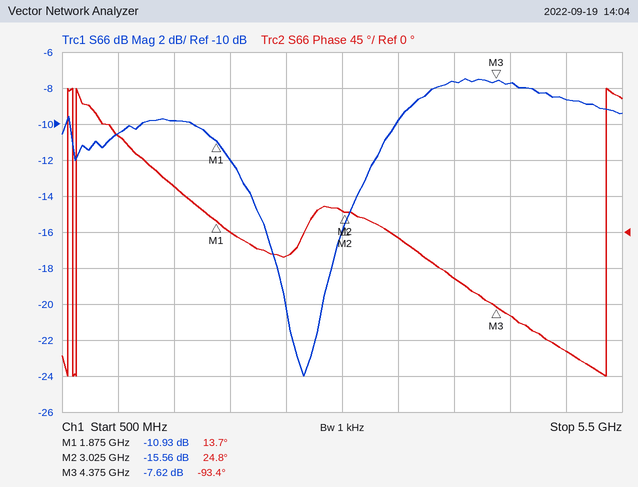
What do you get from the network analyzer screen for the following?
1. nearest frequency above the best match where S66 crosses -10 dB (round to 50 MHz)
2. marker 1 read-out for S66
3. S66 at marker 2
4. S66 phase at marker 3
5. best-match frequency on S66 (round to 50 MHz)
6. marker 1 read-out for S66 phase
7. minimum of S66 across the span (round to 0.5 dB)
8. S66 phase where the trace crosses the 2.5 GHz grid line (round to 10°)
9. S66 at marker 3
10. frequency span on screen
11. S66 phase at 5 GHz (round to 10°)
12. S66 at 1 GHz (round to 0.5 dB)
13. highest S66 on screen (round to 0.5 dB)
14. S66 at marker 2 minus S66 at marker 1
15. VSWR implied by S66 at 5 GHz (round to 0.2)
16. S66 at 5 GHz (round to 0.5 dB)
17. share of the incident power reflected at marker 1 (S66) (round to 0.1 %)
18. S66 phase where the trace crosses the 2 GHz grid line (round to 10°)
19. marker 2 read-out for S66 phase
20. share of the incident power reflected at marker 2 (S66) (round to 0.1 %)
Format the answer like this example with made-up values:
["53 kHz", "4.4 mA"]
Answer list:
["3.50 GHz", "-10.93 dB", "-15.56 dB", "-93.4°", "2.65 GHz", "13.7°", "-24.0 dB", "-30°", "-7.62 dB", "5 GHz", "-150°", "-10.5 dB", "-7.5 dB", "-4.63 dB", "2.2", "-8.5 dB", "8.1 %", "0°", "24.8°", "2.8 %"]
